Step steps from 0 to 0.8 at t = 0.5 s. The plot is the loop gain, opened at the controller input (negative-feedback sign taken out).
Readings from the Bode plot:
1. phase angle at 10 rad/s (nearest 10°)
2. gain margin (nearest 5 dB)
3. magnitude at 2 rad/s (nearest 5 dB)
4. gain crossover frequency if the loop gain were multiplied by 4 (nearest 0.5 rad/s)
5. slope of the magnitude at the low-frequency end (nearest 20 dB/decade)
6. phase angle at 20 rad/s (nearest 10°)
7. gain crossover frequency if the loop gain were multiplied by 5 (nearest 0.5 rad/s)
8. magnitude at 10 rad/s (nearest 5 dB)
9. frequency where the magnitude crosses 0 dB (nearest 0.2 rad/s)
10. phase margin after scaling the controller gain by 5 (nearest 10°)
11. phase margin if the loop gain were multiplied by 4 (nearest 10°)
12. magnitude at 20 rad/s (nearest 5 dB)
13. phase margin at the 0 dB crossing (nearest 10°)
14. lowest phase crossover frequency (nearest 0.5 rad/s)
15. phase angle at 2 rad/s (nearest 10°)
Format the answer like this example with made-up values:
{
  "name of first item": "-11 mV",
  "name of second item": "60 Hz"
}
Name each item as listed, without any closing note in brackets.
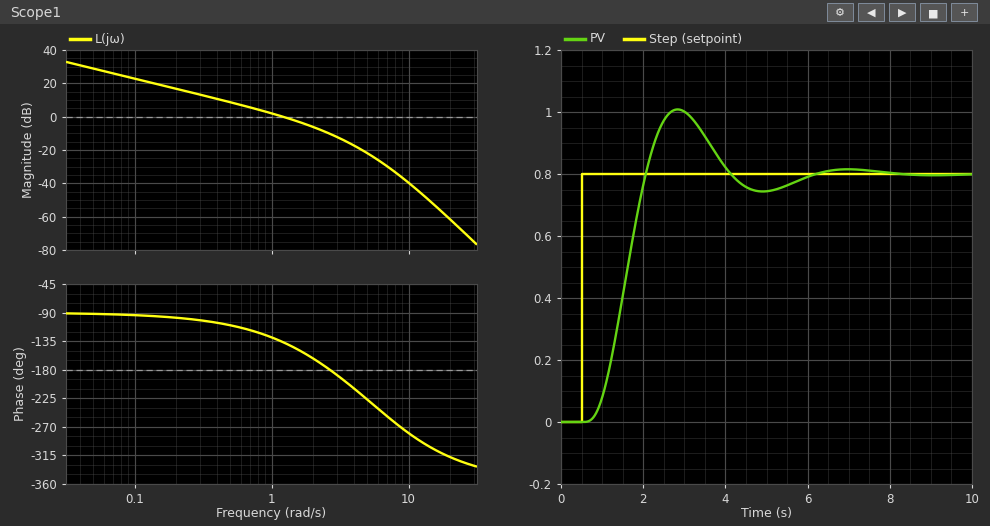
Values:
{
  "phase angle at 10 rad/s": "-280°",
  "gain margin": "10 dB",
  "magnitude at 2 rad/s": "-5 dB",
  "gain crossover frequency if the loop gain were multiplied by 4": "3.0 rad/s",
  "slope of the magnitude at the low-frequency end": "-20 dB/decade",
  "phase angle at 20 rad/s": "-320°",
  "gain crossover frequency if the loop gain were multiplied by 5": "3.5 rad/s",
  "magnitude at 10 rad/s": "-40 dB",
  "frequency where the magnitude crosses 0 dB": "1.2 rad/s",
  "phase margin after scaling the controller gain by 5": "-20°",
  "phase margin if the loop gain were multiplied by 4": "-10°",
  "magnitude at 20 rad/s": "-60 dB",
  "phase margin at the 0 dB crossing": "40°",
  "lowest phase crossover frequency": "2.5 rad/s",
  "phase angle at 2 rad/s": "-160°"
}
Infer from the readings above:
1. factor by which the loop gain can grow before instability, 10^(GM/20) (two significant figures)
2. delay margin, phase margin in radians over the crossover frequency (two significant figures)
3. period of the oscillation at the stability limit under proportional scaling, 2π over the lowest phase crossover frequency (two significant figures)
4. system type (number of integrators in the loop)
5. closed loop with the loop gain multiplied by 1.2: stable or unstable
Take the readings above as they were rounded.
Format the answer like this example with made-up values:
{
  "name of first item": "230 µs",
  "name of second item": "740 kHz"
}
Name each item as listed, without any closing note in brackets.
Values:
{
  "factor by which the loop gain can grow before instability, 10^(GM/20)": "3.2",
  "delay margin, phase margin in radians over the crossover frequency": "0.58 s",
  "period of the oscillation at the stability limit under proportional scaling, 2π over the lowest phase crossover frequency": "2.5 s",
  "system type": "1",
  "closed loop with the loop gain multiplied by 1.2: stable or unstable": "stable"
}
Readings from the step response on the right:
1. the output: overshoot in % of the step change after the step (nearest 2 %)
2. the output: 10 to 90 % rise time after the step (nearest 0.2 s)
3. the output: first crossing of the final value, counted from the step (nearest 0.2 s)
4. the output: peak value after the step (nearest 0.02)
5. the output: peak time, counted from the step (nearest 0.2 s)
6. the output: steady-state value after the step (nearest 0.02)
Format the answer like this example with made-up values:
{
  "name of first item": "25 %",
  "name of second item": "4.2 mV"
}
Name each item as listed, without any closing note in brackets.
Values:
{
  "the output: overshoot in % of the step change after the step": "26 %",
  "the output: 10 to 90 % rise time after the step": "1.0 s",
  "the output: first crossing of the final value, counted from the step": "1.6 s",
  "the output: peak value after the step": "1.00",
  "the output: peak time, counted from the step": "2.4 s",
  "the output: steady-state value after the step": "0.80"
}
